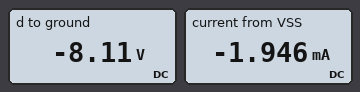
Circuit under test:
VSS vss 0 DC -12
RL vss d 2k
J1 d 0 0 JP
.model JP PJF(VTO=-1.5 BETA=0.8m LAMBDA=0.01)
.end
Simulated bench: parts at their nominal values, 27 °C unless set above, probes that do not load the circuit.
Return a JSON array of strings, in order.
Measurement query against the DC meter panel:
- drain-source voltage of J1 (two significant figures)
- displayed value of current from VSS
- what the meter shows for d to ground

["-8.1 V", "-1.946 mA", "-8.11 V"]
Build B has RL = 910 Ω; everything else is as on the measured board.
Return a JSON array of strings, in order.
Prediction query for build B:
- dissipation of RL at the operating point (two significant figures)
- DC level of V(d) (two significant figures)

["3.6 mW", "-10 V"]
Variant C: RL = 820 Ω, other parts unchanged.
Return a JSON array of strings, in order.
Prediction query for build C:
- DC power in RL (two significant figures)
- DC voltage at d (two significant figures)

["3.2 mW", "-10 V"]
